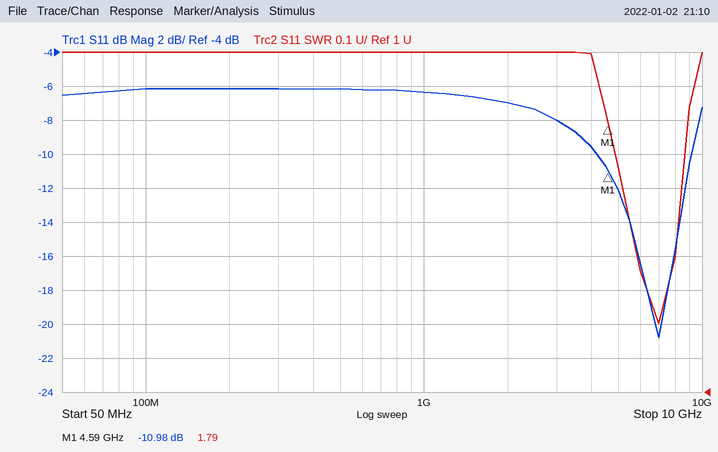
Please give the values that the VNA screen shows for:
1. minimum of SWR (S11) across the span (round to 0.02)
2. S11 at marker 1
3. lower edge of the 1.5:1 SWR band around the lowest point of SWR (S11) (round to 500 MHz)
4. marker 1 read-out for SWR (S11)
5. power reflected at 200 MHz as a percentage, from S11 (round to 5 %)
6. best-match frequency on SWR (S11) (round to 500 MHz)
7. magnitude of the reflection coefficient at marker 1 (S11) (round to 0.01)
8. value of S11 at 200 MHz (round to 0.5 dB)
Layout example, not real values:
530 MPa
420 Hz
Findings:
1.20
-10.98 dB
5.5 GHz
1.79
25 %
7.0 GHz
0.28
-6.0 dB
